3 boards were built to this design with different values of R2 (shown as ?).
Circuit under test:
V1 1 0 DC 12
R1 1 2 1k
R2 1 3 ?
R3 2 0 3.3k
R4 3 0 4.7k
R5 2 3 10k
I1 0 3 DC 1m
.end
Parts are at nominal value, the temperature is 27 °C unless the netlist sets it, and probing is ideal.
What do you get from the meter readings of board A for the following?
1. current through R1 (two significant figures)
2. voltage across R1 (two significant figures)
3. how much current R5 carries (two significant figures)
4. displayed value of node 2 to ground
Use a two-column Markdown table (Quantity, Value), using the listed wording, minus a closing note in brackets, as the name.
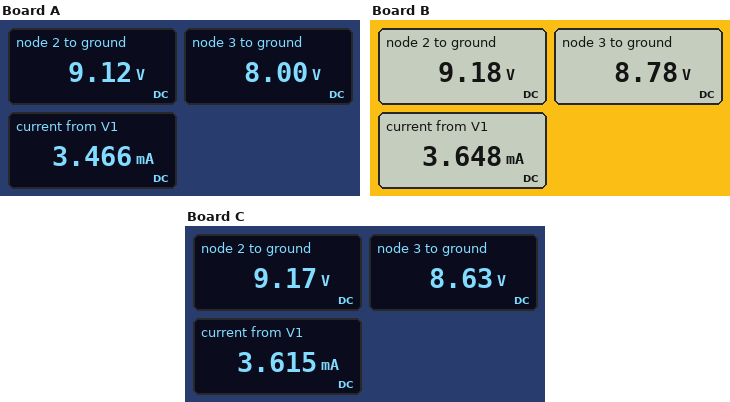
| Quantity | Value |
|---|---|
| current through R1 | 2.9 mA |
| voltage across R1 | 2.9 V |
| how much current R5 carries | 110 µA |
| displayed value of node 2 to ground | 9.12 V |
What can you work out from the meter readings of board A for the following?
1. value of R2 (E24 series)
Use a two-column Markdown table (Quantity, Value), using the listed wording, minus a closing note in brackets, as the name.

| Quantity | Value |
|---|---|
| value of R2 | 6.8 kΩ |
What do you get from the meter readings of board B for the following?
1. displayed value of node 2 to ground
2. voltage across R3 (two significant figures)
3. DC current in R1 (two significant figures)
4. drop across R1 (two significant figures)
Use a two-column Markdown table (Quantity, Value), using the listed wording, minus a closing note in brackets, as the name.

| Quantity | Value |
|---|---|
| displayed value of node 2 to ground | 9.18 V |
| voltage across R3 | 9.2 V |
| DC current in R1 | 2.8 mA |
| drop across R1 | 2.8 V |
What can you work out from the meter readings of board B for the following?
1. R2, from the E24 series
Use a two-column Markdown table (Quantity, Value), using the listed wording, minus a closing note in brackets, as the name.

| Quantity | Value |
|---|---|
| R2, from the E24 series | 3.9 kΩ |
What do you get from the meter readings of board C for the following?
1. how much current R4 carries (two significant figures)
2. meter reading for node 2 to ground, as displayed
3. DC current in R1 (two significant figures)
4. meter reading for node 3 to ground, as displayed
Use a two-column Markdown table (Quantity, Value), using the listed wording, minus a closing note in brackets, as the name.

| Quantity | Value |
|---|---|
| how much current R4 carries | 1.8 mA |
| meter reading for node 2 to ground, as displayed | 9.17 V |
| DC current in R1 | 2.8 mA |
| meter reading for node 3 to ground, as displayed | 8.63 V |
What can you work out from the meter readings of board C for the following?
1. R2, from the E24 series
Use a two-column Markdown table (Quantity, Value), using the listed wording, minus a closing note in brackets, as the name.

| Quantity | Value |
|---|---|
| R2, from the E24 series | 4.3 kΩ |
